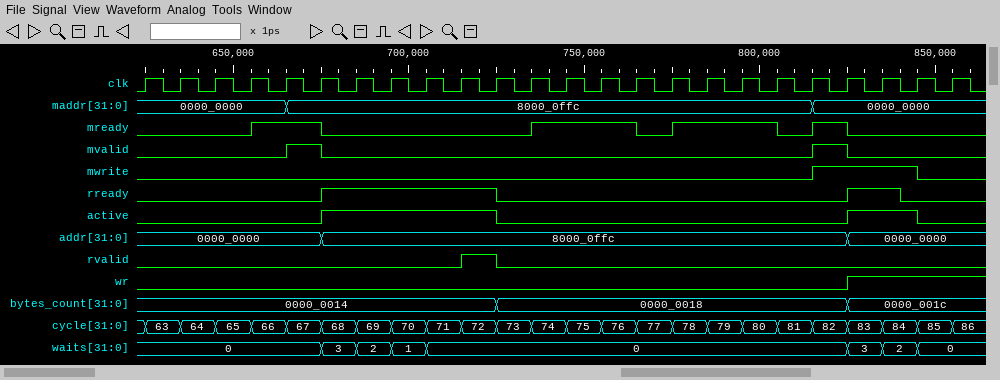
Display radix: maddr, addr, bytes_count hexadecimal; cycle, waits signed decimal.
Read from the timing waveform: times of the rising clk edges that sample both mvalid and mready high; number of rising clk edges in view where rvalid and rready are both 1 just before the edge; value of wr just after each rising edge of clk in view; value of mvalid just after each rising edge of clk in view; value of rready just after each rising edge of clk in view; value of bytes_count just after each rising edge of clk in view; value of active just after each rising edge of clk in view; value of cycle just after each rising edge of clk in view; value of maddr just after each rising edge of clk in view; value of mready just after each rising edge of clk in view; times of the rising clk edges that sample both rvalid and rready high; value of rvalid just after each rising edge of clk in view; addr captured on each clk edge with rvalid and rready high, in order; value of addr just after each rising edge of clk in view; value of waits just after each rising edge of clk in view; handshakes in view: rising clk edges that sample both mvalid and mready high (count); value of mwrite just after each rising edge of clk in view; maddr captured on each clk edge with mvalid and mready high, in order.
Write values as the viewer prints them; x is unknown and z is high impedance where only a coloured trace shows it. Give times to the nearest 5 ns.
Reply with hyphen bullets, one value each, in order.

- 675 ns, 825 ns
- 1
- 0 0 0 0 0 0 0 0 0 0 0 0 0 0 0 0 0 0 0 0 1 1 1 1
- 0 0 0 0 1 0 0 0 0 0 0 0 0 0 0 0 0 0 0 1 0 0 0 0
- 0 0 0 0 0 1 1 1 1 1 0 0 0 0 0 0 0 0 0 0 1 1 0 0
- 0000_0014, 0000_0014, 0000_0014, 0000_0014, 0000_0014, 0000_0014, 0000_0014, 0000_0014, 0000_0014, 0000_0014, 0000_0018, 0000_0018, 0000_0018, 0000_0018, 0000_0018, 0000_0018, 0000_0018, 0000_0018, 0000_0018, 0000_0018, 0000_001c, 0000_001c, 0000_001c, 0000_001c
- 0 0 0 0 0 1 1 1 1 1 0 0 0 0 0 0 0 0 0 0 1 1 0 0
- 63, 64, 65, 66, 67, 68, 69, 70, 71, 72, 73, 74, 75, 76, 77, 78, 79, 80, 81, 82, 83, 84, 85, 86
- 0000_0000, 0000_0000, 0000_0000, 0000_0000, 8000_0ffc, 8000_0ffc, 8000_0ffc, 8000_0ffc, 8000_0ffc, 8000_0ffc, 8000_0ffc, 8000_0ffc, 8000_0ffc, 8000_0ffc, 8000_0ffc, 8000_0ffc, 8000_0ffc, 8000_0ffc, 8000_0ffc, 0000_0000, 0000_0000, 0000_0000, 0000_0000, 0000_0000
- 0 0 0 1 1 0 0 0 0 0 0 1 1 1 0 1 1 1 0 1 0 0 0 0
- 725 ns
- 0 0 0 0 0 0 0 0 0 1 0 0 0 0 0 0 0 0 0 0 0 0 0 0
- 8000_0ffc
- 0000_0000, 0000_0000, 0000_0000, 0000_0000, 0000_0000, 8000_0ffc, 8000_0ffc, 8000_0ffc, 8000_0ffc, 8000_0ffc, 8000_0ffc, 8000_0ffc, 8000_0ffc, 8000_0ffc, 8000_0ffc, 8000_0ffc, 8000_0ffc, 8000_0ffc, 8000_0ffc, 8000_0ffc, 0000_0000, 0000_0000, 0000_0000, 0000_0000
- 0, 0, 0, 0, 0, 3, 2, 1, 0, 0, 0, 0, 0, 0, 0, 0, 0, 0, 0, 0, 3, 2, 0, 0
- 2
- 0 0 0 0 0 0 0 0 0 0 0 0 0 0 0 0 0 0 0 1 1 1 0 0
- 8000_0ffc, 0000_0000
